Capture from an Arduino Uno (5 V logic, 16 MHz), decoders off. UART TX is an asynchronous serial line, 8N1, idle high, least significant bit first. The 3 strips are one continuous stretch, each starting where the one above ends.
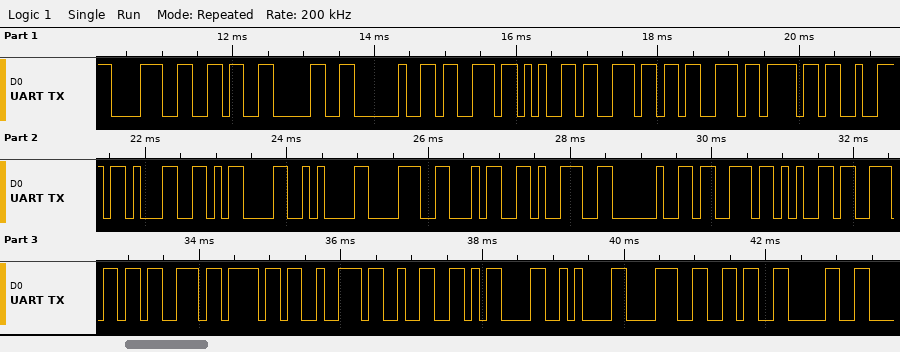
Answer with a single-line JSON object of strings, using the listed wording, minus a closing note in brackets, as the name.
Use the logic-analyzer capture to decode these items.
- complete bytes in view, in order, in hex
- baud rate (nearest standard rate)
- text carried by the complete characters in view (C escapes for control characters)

{"complete bytes in view, in order, in hex": "38 36 30 20 73 65 6E 73 6F 72 31 0D 0A 38 34 39 20 73 65 6E 73 6F 72 32 0D 0A 38 36 30", "baud rate": "9600 baud", "text carried by the complete characters in view": "\"860 sensor1\\r\\n849 sensor2\\r\\n860\""}
